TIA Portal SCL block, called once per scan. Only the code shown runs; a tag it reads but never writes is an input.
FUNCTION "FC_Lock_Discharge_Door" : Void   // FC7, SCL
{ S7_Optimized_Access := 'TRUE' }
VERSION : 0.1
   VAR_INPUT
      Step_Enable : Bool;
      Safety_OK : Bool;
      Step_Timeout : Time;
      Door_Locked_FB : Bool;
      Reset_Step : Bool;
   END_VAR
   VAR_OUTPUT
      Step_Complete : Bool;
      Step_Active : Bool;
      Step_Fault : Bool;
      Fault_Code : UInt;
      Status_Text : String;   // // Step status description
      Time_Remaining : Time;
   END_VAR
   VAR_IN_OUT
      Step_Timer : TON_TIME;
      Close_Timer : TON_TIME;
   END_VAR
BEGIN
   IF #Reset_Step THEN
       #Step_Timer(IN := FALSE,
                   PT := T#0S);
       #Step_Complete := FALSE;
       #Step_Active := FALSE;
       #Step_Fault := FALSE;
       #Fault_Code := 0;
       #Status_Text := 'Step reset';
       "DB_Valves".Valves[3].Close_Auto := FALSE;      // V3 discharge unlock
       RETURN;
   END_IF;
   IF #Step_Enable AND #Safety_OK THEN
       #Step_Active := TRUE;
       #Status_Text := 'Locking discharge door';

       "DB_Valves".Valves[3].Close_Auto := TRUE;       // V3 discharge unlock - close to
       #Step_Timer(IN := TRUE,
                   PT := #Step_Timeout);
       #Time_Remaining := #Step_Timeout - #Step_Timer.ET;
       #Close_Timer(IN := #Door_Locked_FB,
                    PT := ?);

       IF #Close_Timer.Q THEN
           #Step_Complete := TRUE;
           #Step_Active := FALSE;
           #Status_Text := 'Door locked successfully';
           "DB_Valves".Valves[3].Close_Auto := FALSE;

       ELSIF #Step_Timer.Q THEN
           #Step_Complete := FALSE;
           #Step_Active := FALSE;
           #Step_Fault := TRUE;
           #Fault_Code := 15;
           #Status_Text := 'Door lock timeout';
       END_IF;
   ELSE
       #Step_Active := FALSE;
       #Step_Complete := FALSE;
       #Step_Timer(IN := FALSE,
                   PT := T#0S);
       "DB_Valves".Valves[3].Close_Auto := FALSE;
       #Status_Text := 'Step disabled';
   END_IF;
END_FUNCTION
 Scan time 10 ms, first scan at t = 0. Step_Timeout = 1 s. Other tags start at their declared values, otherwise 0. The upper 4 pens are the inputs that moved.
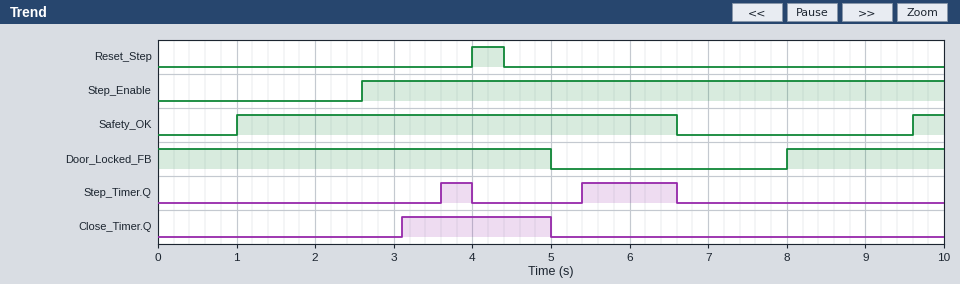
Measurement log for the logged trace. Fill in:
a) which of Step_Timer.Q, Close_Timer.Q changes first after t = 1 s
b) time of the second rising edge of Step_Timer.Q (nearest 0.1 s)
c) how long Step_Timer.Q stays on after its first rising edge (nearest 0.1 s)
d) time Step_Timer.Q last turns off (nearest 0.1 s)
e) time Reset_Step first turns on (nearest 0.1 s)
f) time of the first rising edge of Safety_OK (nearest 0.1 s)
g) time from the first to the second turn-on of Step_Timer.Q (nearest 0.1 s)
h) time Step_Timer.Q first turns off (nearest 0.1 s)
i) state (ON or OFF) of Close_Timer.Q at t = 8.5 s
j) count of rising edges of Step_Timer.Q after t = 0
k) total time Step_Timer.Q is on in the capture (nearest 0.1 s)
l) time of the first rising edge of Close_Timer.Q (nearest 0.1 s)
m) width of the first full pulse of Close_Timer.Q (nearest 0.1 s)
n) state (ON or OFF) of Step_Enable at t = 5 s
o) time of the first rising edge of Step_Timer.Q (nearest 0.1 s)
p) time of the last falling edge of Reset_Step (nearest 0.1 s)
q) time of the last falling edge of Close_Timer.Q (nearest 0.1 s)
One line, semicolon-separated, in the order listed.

Close_Timer.Q; 5.4 s; 0.4 s; 6.6 s; 4.0 s; 1.0 s; 1.8 s; 4.0 s; OFF; 2; 1.6 s; 3.1 s; 1.9 s; ON; 3.6 s; 4.4 s; 5.0 s
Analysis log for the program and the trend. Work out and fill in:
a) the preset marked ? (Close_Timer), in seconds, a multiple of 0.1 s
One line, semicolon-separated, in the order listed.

0.5 s
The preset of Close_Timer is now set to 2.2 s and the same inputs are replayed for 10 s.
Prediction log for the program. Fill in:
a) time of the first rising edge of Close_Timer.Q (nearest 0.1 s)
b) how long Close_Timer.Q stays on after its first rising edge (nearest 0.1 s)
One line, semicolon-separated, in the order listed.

4.8 s; 0.2 s
